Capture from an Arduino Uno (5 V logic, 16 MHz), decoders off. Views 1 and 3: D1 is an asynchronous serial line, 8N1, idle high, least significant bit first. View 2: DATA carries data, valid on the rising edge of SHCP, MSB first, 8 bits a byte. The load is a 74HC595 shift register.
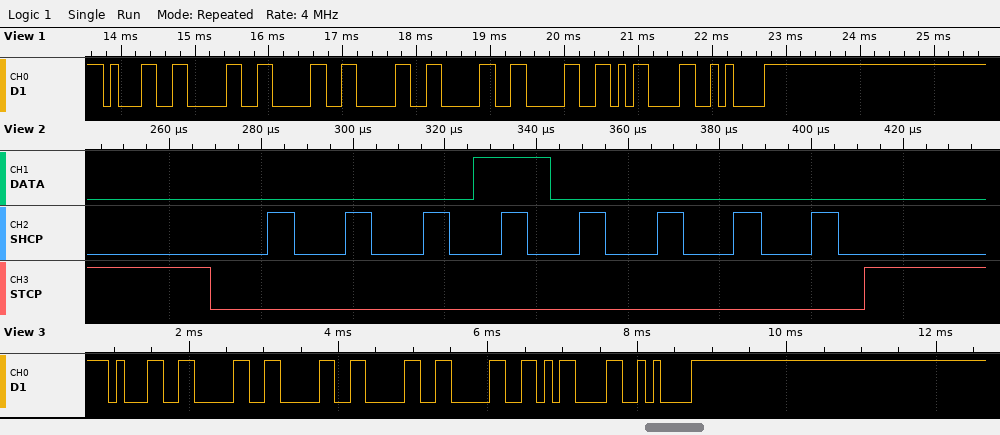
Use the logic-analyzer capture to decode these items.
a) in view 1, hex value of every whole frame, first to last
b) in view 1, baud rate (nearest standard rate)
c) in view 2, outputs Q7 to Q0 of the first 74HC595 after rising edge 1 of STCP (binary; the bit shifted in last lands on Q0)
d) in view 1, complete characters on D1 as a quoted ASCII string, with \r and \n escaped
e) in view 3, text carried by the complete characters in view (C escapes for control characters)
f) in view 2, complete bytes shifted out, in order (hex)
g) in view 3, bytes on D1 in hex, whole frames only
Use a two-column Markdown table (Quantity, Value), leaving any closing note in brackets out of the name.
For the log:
| Quantity | Value |
|---|---|
| in view 1, hex value of every whole frame, first to last | 31 30 30 30 30 30 0D 0A |
| in view 1, baud rate | 9600 baud |
| in view 2, outputs Q7 to Q0 of the first 74HC595 after rising edge 1 of STCP | 00010000 |
| in view 1, complete characters on D1 as a quoted ASCII string, with \r and \n escaped | "100000\r\n" |
| in view 3, text carried by the complete characters in view | "10000\r\n" |
| in view 2, complete bytes shifted out, in order | 10 |
| in view 3, bytes on D1 in hex, whole frames only | 0x31 0x30 0x30 0x30 0x30 0x0D 0x0A |
